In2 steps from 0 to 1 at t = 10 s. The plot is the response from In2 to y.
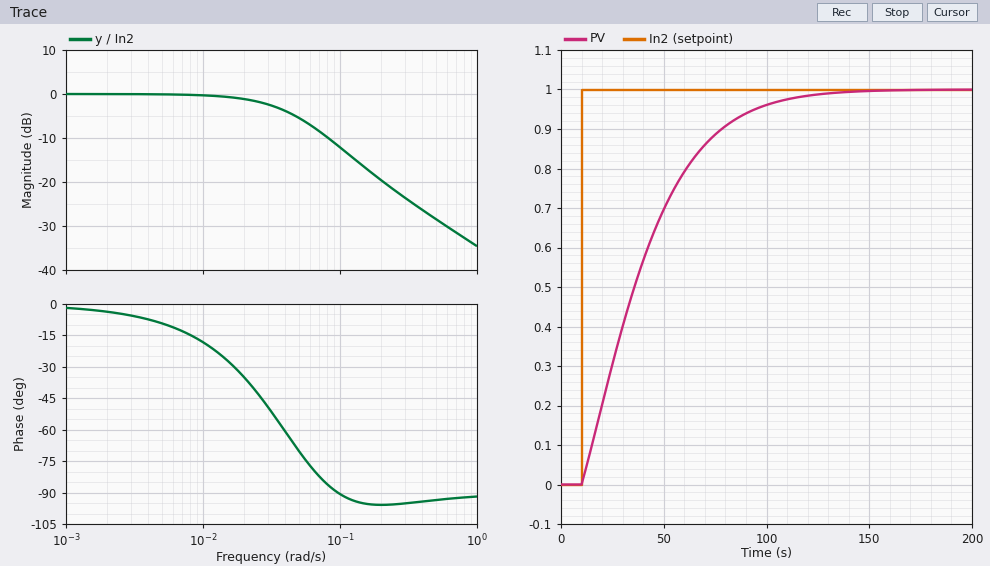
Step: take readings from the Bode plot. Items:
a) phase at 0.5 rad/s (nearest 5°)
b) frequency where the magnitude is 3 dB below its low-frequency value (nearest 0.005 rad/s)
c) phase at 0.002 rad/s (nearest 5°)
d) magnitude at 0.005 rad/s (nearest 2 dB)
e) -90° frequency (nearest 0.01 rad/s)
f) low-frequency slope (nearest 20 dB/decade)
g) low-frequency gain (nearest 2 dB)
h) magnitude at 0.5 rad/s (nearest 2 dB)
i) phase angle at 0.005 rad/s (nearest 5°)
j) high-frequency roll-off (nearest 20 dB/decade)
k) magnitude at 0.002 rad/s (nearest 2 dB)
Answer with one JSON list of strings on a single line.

["-95°", "0.035 rad/s", "-5°", "0 dB", "0.10 rad/s", "0 dB/decade", "0 dB", "-28 dB", "-10°", "-20 dB/decade", "0 dB"]
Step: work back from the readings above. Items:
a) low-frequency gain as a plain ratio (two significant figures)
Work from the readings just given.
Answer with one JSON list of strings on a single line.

["1.0"]
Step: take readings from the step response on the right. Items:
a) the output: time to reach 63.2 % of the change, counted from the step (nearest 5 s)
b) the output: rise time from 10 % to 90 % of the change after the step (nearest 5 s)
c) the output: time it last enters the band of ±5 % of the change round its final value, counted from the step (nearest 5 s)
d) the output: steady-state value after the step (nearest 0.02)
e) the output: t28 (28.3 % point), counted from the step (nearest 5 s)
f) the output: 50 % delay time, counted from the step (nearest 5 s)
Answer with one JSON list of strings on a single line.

["35 s", "65 s", "85 s", "1.00", "15 s", "25 s"]
